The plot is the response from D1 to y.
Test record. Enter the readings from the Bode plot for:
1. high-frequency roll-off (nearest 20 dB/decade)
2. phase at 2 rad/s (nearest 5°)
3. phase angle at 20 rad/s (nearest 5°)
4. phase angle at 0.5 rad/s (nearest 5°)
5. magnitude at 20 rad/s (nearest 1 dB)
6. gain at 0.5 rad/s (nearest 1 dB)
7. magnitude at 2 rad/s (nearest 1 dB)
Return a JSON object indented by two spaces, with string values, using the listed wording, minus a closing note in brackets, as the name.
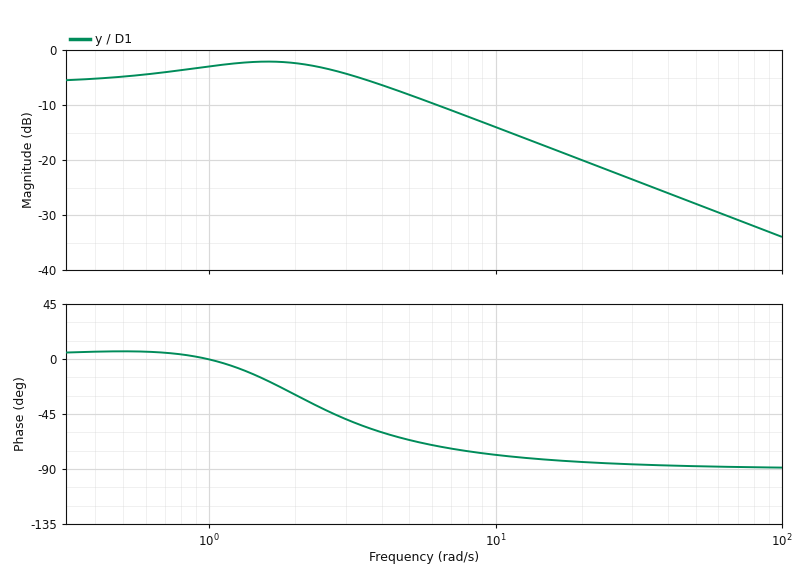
{
  "high-frequency roll-off": "-20 dB/decade",
  "phase at 2 rad/s": "-30°",
  "phase angle at 20 rad/s": "-85°",
  "phase angle at 0.5 rad/s": "5°",
  "magnitude at 20 rad/s": "-20 dB",
  "gain at 0.5 rad/s": "-5 dB",
  "magnitude at 2 rad/s": "-2 dB"
}
